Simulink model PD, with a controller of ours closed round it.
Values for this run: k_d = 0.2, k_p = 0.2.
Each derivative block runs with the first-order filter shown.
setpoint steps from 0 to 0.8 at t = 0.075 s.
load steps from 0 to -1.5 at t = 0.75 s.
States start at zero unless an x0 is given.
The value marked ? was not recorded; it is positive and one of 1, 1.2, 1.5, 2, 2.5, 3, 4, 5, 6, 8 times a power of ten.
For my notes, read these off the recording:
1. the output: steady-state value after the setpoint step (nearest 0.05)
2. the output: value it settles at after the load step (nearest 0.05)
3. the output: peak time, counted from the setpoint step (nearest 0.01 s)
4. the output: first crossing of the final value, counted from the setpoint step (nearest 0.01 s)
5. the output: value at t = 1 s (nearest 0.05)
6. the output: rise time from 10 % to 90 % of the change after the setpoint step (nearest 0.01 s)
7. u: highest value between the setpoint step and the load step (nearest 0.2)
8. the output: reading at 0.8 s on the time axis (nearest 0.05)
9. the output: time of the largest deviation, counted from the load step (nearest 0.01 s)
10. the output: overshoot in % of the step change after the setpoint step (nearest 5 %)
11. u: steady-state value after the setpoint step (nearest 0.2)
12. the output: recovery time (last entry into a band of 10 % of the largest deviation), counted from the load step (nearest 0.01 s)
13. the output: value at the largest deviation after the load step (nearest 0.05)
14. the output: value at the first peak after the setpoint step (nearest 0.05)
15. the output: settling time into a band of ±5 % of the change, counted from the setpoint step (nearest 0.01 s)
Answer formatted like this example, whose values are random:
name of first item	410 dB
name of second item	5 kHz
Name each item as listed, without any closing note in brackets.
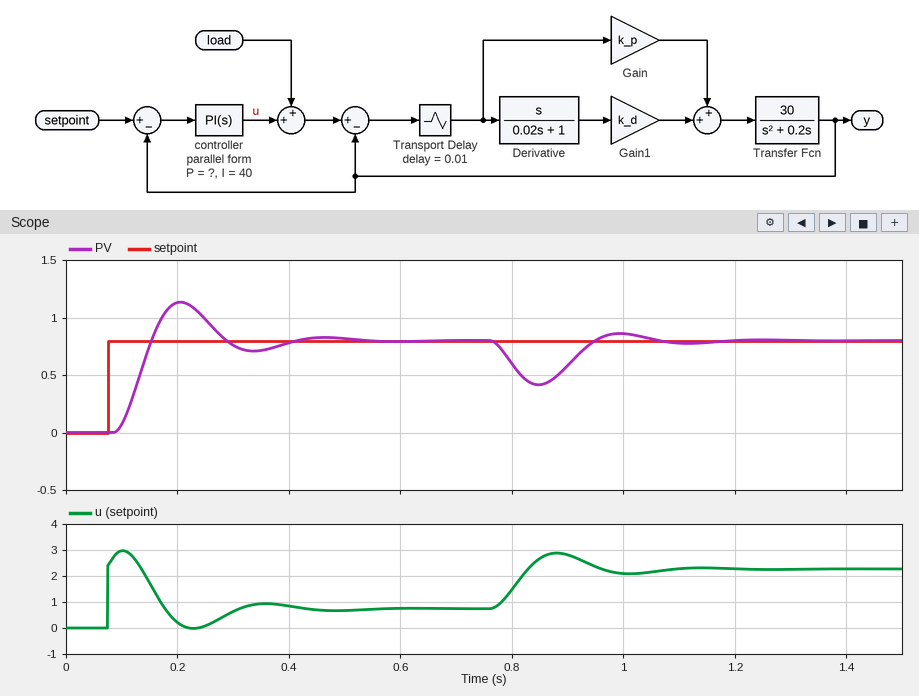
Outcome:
the output: steady-state value after the setpoint step	0.80
the output: value it settles at after the load step	0.80
the output: peak time, counted from the setpoint step	0.13 s
the output: first crossing of the final value, counted from the setpoint step	0.08 s
the output: value at t = 1 s	0.85
the output: rise time from 10 % to 90 % of the change after the setpoint step	0.05 s
u: highest value between the setpoint step and the load step	3.0
the output: reading at 0.8 s on the time axis	0.60
the output: time of the largest deviation, counted from the load step	0.10 s
the output: overshoot in % of the step change after the setpoint step	40 %
u: steady-state value after the setpoint step	0.8
the output: recovery time (last entry into a band of 10 % of the largest deviation), counted from the load step	0.28 s
the output: value at the largest deviation after the load step	0.40
the output: value at the first peak after the setpoint step	1.15
the output: settling time into a band of ±5 % of the change, counted from the setpoint step	0.31 s
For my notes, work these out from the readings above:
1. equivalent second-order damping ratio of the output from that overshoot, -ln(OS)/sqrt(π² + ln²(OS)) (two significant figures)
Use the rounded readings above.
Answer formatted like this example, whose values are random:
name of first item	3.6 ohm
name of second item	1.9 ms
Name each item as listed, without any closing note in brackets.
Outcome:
equivalent second-order damping ratio of the output from that overshoot, -ln(OS)/sqrt(π² + ln²(OS))	0.28
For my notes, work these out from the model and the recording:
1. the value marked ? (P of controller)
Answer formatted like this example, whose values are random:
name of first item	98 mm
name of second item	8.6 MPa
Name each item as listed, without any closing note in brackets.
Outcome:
the value marked ?	3
